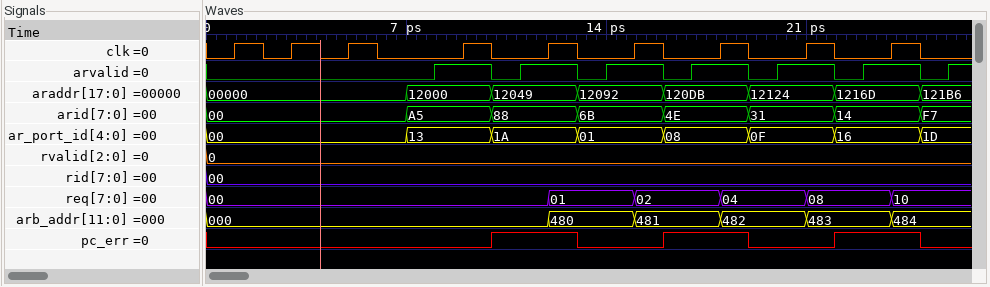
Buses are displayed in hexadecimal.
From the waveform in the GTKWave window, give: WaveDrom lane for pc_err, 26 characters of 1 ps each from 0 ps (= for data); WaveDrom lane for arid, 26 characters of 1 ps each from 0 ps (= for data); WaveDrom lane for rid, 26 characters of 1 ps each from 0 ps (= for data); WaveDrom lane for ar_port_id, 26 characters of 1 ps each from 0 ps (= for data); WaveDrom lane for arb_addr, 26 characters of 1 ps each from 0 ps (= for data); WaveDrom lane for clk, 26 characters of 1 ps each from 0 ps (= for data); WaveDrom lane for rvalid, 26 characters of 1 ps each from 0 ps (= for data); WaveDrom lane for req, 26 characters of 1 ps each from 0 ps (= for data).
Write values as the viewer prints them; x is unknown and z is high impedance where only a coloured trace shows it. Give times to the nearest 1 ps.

{name: 'pc_err', wave: '0.........1..0..1..0..1..0'}
{name: 'arid', wave: '=......=..=..=..=..=..=..=', data: '00 A5 88 6B 4E 31 14 F7'}
{name: 'rid', wave: '=.........................', data: '00'}
{name: 'ar_port_id', wave: '=......=..=..=..=..=..=..=', data: '00 13 1A 01 08 0F 16 1D'}
{name: 'arb_addr', wave: '=...........=..=..=..=..=.', data: '000 480 481 482 483 484'}
{name: 'clk', wave: '0101010..10.10.10.10.10.10'}
{name: 'rvalid', wave: '=.........................', data: '0'}
{name: 'req', wave: '=...........=..=..=..=..=.', data: '00 01 02 04 08 10'}
